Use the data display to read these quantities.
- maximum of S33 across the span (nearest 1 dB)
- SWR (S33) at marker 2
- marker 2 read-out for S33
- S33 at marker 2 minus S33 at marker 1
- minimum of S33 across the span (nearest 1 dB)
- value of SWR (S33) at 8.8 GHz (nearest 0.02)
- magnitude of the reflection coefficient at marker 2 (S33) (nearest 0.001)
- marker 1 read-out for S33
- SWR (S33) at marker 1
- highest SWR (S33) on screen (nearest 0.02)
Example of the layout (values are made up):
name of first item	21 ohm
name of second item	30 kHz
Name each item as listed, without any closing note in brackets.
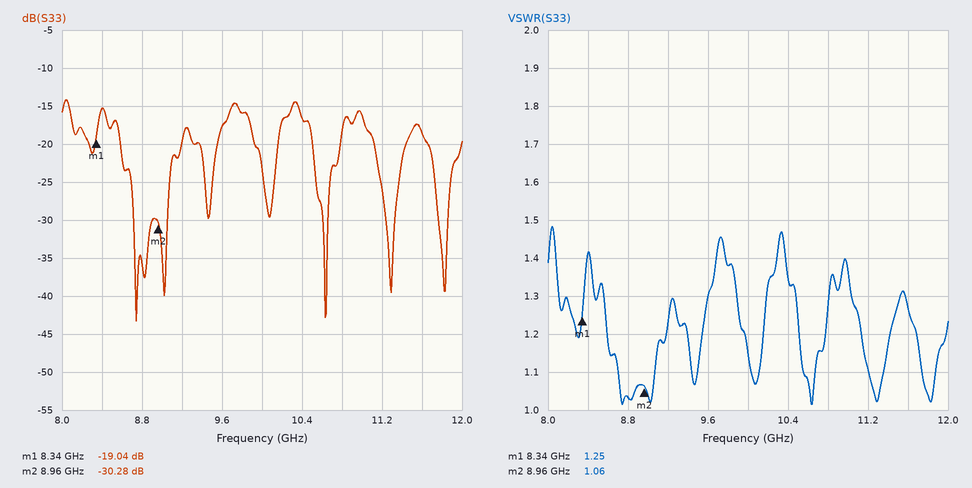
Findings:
maximum of S33 across the span	-14 dB
SWR (S33) at marker 2	1.06
marker 2 read-out for S33	-30.28 dB
S33 at marker 2 minus S33 at marker 1	-11.24 dB
minimum of S33 across the span	-43 dB
value of SWR (S33) at 8.8 GHz	1.04
magnitude of the reflection coefficient at marker 2 (S33)	0.031
marker 1 read-out for S33	-19.04 dB
SWR (S33) at marker 1	1.25
highest SWR (S33) on screen	1.48
